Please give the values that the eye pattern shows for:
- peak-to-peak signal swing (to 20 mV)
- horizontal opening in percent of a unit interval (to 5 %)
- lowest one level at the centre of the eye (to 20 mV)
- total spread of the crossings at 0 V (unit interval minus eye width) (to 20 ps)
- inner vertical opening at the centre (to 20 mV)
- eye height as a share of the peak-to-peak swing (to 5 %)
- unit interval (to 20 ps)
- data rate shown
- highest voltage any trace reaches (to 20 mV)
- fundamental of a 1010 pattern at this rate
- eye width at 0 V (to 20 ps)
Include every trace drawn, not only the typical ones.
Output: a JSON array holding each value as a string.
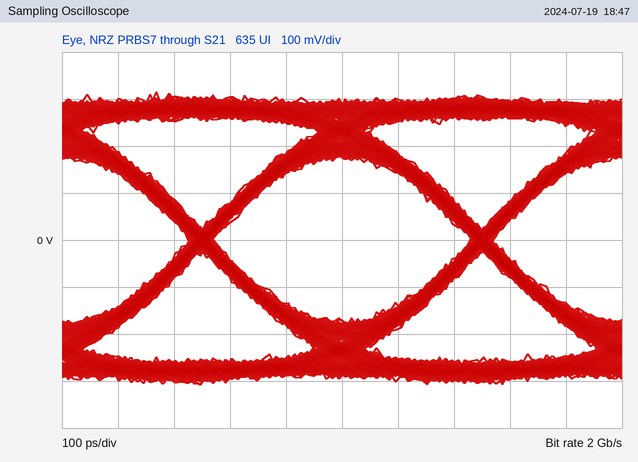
["620 mV", "90 %", "180 mV", "40 ps", "340 mV", "55 %", "500 ps", "2 Gb/s", "320 mV", "1 GHz", "460 ps"]
